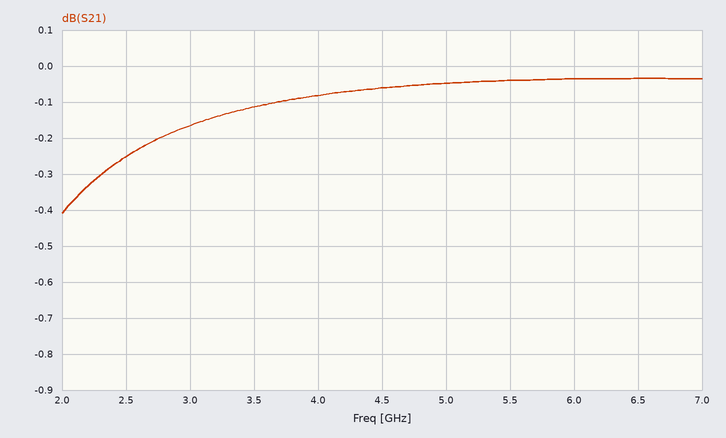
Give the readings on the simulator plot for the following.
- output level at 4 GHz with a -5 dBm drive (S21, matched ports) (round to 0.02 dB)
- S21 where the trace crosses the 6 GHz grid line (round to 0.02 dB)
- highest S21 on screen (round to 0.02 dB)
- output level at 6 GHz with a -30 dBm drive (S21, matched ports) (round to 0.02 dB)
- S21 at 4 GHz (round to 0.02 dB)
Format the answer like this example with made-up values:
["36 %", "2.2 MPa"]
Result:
["-5.08 dBm", "-0.04 dB", "-0.04 dB", "-30.04 dBm", "-0.08 dB"]
